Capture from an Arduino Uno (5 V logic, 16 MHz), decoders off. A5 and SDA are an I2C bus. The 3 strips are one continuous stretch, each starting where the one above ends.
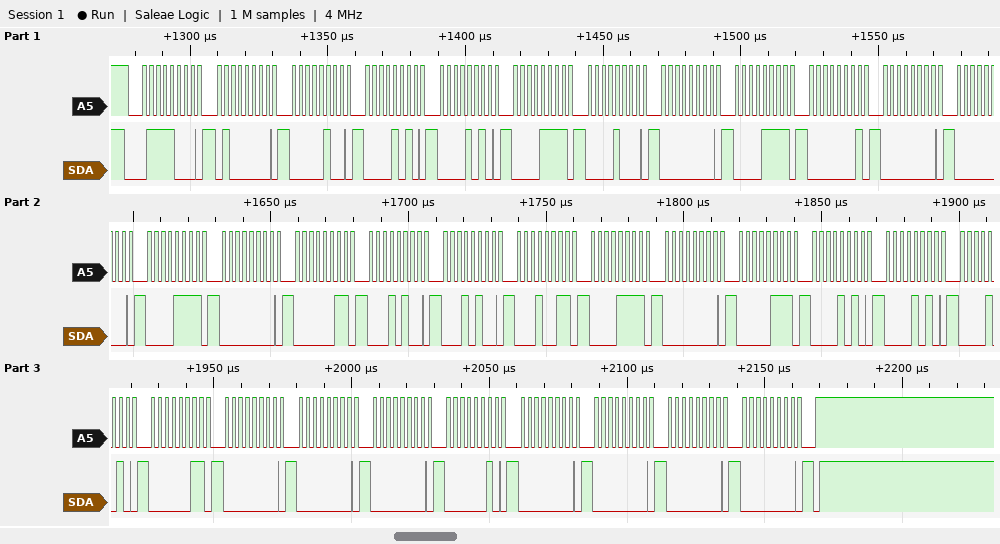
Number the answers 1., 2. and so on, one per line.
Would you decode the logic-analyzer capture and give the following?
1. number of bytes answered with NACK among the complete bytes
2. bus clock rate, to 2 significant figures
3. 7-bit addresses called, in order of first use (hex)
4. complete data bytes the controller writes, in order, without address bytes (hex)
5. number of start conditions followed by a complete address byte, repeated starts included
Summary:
1. 0
2. 400 kHz
3. 0x3C
4. 40 04 0A 0A 0F 08 00 0F 01 00 00 0F 00 03 14 14 13 0F 00 07 0A 0A 0A 03 00 00 00 02 00 00 00 00
5. 1
